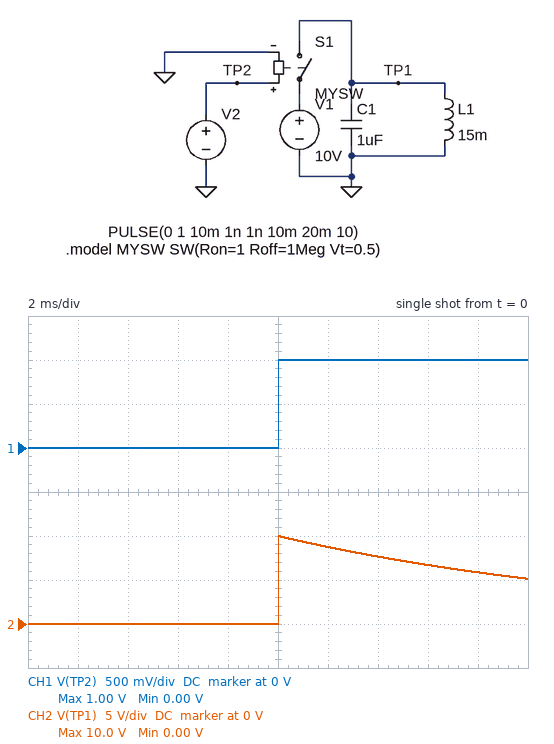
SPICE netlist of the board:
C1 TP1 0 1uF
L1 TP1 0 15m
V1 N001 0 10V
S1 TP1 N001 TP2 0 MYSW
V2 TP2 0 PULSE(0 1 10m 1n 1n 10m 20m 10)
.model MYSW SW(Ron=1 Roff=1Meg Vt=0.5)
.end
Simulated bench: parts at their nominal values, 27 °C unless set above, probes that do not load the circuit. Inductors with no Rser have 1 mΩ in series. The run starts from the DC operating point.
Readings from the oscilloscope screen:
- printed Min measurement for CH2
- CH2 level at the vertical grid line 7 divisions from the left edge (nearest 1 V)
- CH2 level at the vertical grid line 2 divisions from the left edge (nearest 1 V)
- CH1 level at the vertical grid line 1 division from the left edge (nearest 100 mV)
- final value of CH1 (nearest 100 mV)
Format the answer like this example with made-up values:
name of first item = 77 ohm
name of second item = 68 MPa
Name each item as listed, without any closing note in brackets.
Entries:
printed Min measurement for CH2 = 0.00 V
CH2 level at the vertical grid line 7 divisions from the left edge = 8 V
CH2 level at the vertical grid line 2 divisions from the left edge = 0 V
CH1 level at the vertical grid line 1 division from the left edge = 0 V
final value of CH1 = 1.0 V
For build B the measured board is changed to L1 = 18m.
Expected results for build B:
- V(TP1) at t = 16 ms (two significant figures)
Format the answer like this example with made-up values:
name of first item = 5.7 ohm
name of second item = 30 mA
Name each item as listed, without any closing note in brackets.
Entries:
V(TP1) at t = 16 ms = 7.2 V
